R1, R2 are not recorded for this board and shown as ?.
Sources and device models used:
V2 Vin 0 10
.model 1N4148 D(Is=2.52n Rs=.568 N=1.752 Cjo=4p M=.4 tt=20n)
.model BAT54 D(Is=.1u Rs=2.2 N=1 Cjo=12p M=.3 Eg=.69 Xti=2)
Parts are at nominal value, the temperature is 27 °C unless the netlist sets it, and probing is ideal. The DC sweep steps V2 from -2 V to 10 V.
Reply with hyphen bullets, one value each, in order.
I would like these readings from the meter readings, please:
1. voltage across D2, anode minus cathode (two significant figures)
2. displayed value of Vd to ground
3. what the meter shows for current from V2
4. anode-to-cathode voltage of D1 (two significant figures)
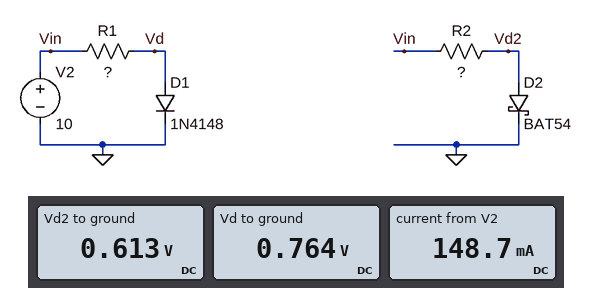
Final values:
- 610 mV
- 0.764 V
- 148.7 mA
- 760 mV
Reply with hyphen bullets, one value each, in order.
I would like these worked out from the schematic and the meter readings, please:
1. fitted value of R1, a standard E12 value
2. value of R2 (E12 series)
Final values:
- 270 Ω
- 82 Ω
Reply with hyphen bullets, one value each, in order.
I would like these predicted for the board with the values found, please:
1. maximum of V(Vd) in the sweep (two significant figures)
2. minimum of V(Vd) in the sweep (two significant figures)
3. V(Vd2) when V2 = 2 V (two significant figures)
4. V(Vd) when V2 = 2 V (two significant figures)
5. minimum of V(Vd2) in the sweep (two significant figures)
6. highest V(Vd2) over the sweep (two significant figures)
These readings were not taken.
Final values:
- 760 mV
- -2.0 V
- 360 mV
- 660 mV
- -2.0 V
- 610 mV
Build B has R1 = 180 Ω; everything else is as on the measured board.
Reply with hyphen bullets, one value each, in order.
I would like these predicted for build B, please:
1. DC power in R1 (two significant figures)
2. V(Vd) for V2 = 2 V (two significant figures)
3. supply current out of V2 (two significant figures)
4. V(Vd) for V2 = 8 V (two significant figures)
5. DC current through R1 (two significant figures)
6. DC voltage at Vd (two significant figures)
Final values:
- 470 mW
- 680 mV
- 170 mA
- 770 mV
- 51 mA
- 790 mV
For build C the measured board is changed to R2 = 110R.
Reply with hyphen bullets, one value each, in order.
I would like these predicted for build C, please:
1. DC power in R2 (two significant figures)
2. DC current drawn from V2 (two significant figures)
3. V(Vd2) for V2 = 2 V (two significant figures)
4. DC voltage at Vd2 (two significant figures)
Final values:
- 810 mW
- 120 mA
- 340 mV
- 540 mV
